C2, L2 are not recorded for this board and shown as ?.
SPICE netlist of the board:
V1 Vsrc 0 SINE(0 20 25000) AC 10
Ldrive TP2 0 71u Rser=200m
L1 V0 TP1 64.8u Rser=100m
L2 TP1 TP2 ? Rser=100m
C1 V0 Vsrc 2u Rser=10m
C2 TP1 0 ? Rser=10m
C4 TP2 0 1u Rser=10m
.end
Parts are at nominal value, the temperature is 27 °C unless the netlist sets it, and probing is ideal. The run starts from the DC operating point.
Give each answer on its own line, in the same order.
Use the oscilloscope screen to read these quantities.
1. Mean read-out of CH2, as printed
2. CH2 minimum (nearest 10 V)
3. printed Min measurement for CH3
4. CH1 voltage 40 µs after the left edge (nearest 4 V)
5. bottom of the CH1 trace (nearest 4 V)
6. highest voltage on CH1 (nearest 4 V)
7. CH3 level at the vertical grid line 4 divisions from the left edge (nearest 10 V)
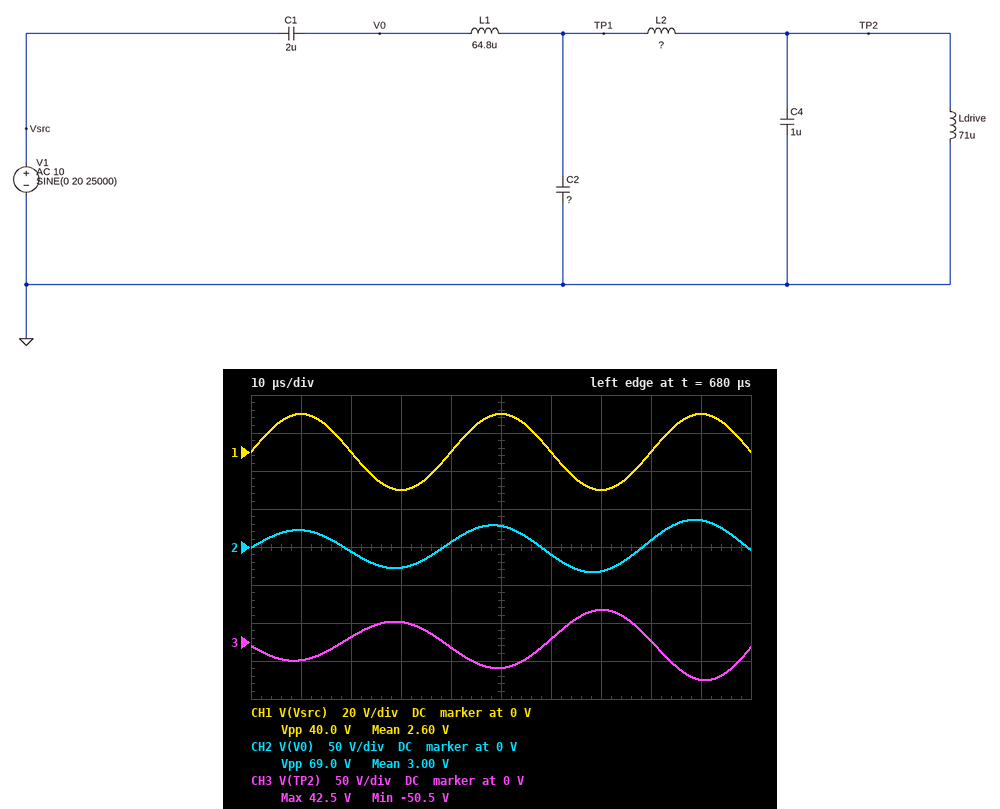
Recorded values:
3.00 V
-30 V
-50.5 V
0 V
-20 V
20 V
-10 V
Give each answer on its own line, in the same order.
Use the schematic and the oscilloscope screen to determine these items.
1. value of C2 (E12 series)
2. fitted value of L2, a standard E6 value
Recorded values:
1.5 µF
100 µH
